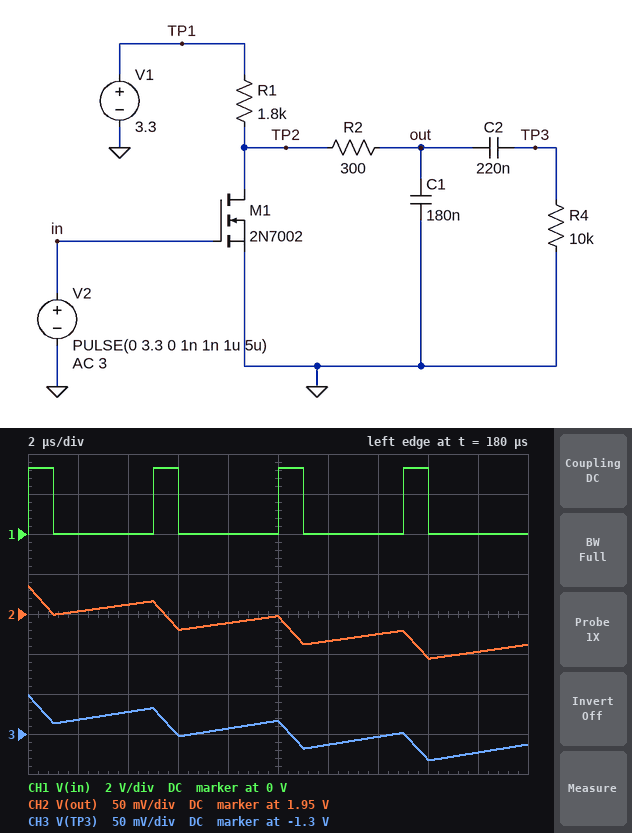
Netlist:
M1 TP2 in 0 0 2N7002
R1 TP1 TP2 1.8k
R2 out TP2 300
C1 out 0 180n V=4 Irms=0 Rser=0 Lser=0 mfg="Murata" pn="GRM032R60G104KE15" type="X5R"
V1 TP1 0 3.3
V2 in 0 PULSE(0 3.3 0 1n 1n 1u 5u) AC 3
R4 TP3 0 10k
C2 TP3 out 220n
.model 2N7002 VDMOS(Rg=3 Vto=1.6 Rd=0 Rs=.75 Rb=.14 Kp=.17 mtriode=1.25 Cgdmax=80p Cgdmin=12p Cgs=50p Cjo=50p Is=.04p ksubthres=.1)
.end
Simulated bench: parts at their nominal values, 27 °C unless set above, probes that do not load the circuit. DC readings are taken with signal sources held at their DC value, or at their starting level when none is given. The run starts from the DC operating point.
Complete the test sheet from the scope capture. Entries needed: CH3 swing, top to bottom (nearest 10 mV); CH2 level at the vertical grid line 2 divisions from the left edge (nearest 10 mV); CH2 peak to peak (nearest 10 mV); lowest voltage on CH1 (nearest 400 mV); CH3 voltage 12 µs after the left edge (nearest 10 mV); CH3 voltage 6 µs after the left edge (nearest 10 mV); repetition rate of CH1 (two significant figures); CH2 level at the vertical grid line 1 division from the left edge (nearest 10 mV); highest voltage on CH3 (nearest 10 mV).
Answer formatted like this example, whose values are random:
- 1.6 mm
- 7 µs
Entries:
- 80 mV
- 1.96 V
- 90 mV
- 0 V
- -1.31 V
- -1.30 V
- 200 kHz
- 1.95 V
- -1.25 V
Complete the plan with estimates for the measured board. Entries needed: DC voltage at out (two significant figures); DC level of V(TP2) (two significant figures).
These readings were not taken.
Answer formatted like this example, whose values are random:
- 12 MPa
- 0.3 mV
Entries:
- 3.3 V
- 3.3 V
